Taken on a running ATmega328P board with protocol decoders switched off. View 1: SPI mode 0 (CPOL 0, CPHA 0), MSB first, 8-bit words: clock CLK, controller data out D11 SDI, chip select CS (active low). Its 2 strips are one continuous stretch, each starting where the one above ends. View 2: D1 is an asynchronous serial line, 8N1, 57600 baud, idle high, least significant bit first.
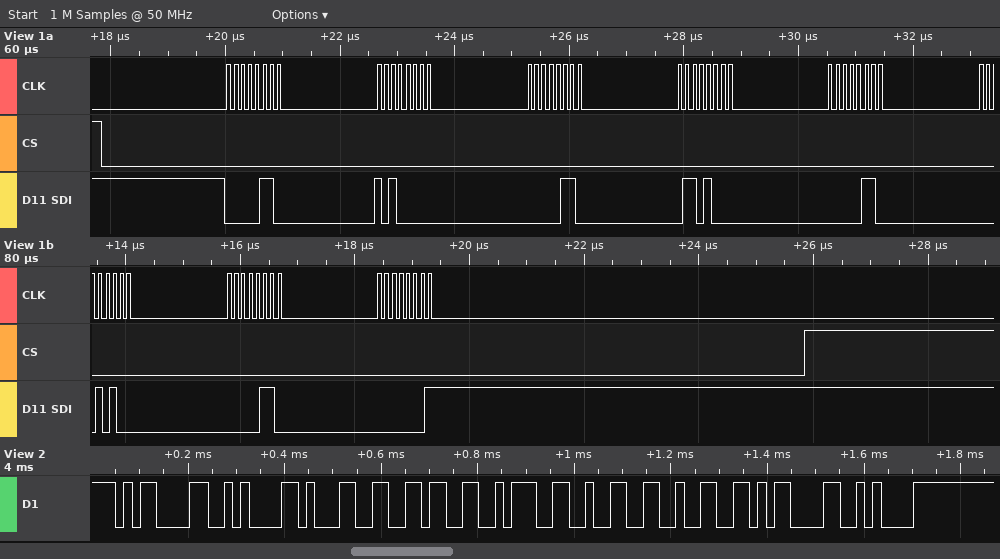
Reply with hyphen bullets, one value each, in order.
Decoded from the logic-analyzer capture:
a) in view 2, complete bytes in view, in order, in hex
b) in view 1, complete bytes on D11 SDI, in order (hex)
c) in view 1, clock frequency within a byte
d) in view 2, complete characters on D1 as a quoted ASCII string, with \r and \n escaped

- 0D 0A 31 36 3A 32 32 0D 0A
- 06 A0 06 68 06 14 06 01
- 8 MHz
- "\r\n16:22\r\n"
